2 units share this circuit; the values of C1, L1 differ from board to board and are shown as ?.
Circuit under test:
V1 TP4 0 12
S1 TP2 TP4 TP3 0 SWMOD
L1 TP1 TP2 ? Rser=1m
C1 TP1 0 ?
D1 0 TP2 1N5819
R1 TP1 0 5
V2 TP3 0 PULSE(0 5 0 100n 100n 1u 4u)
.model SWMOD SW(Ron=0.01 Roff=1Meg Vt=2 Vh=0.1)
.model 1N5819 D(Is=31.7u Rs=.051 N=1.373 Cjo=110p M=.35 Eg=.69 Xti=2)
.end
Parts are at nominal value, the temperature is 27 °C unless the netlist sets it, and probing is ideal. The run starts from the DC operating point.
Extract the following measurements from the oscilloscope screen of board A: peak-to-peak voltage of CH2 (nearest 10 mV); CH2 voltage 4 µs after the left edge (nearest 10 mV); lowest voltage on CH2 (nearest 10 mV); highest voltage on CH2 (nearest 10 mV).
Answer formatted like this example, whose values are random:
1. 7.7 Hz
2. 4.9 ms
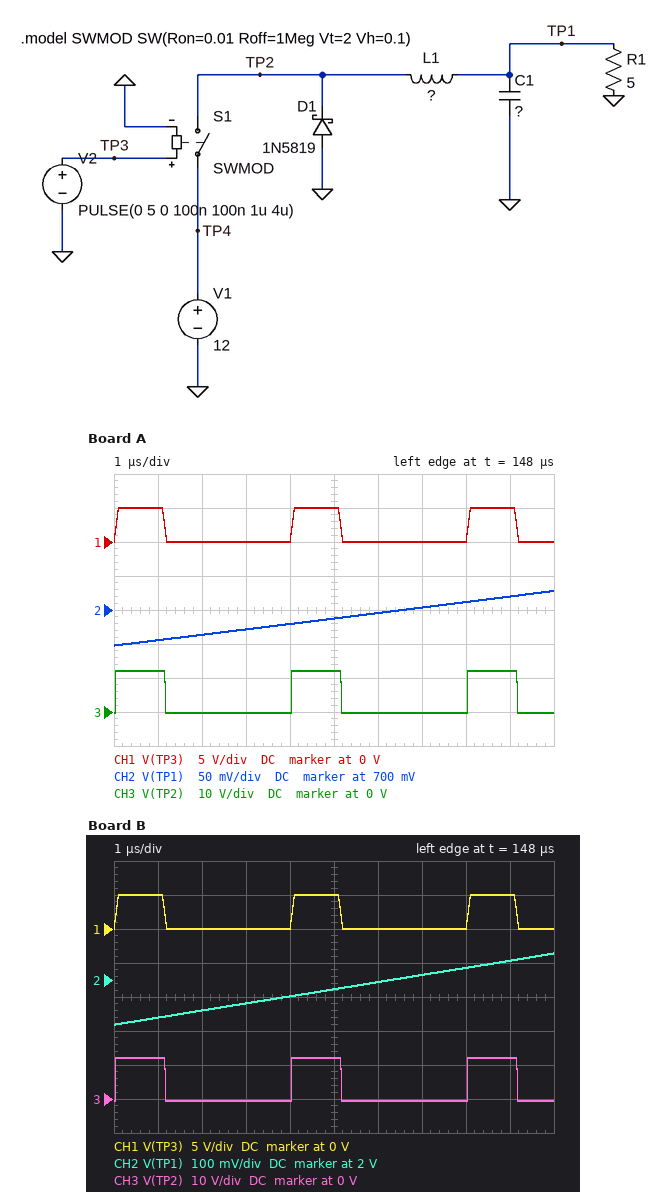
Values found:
1. 80 mV
2. 680 mV
3. 650 mV
4. 730 mV
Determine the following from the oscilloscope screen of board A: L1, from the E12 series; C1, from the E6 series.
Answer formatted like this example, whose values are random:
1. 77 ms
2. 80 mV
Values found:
1. 470 µH
2. 100 µF
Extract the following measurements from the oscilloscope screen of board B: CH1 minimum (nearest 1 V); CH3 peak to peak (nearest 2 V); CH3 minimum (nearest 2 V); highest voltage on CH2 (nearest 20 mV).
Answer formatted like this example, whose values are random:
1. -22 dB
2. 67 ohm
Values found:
1. 0 V
2. 12 V
3. 0 V
4. 2.08 V
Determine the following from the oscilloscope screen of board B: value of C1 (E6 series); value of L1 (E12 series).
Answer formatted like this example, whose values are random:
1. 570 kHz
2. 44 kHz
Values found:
1. 150 µF
2. 100 µH
